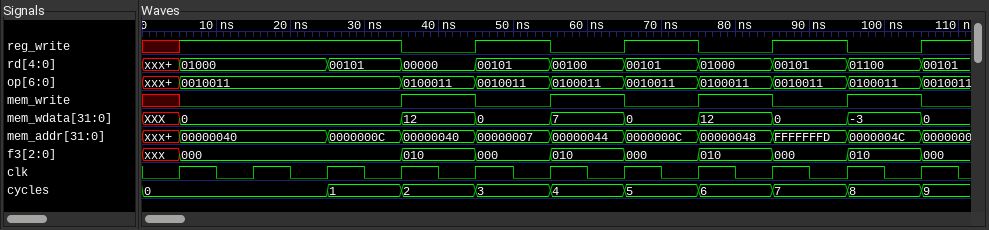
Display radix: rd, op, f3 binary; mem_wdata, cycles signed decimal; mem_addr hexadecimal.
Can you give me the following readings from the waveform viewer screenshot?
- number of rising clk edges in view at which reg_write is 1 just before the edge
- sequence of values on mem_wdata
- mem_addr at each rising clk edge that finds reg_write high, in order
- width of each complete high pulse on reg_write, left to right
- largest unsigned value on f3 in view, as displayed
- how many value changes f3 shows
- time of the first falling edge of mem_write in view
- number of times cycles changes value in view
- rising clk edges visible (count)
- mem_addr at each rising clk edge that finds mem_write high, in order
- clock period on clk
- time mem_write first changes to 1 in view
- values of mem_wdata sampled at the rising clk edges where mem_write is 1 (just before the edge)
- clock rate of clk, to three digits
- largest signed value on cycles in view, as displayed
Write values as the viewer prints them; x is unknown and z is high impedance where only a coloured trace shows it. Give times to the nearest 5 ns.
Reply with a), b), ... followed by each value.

a) 6
b) XXX, 0, 12, 0, 7, 0, 12, 0, -3, 0
c) 00000040, 00000040, 0000000C, 00000007, 0000000C, FFFFFFFD
d) 10 ns, 10 ns, 10 ns
e) 010
f) 9
g) 45 ns
h) 9
i) 11
j) 00000040, 00000044, 00000048, 0000004C
k) 10 ns
l) 35 ns
m) 12, 7, 12, -3
n) 100 MHz
o) 9
